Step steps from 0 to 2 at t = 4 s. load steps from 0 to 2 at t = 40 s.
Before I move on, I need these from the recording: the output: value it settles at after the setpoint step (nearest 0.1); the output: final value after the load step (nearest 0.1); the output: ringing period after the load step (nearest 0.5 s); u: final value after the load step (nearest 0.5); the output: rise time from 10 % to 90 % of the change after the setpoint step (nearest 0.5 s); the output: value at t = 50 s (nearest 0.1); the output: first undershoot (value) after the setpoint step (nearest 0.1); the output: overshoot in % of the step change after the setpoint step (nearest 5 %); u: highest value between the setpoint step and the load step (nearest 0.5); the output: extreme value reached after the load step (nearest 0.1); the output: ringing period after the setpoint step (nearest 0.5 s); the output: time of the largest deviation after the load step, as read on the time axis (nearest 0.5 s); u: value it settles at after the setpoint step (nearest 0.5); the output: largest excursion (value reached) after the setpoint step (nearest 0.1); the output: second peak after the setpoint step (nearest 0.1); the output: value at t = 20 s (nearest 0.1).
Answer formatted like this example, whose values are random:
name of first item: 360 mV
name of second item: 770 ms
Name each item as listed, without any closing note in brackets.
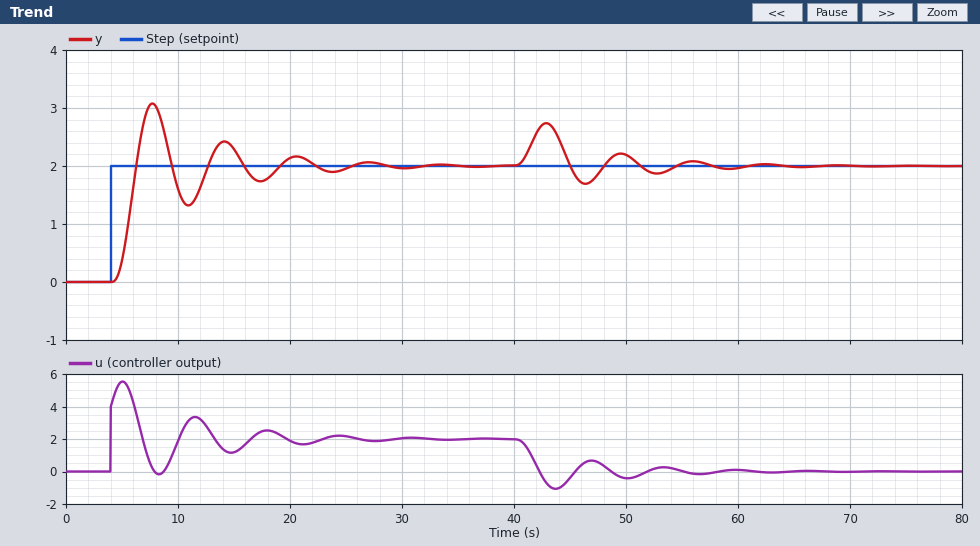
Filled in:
the output: value it settles at after the setpoint step: 2.0
the output: final value after the load step: 2.0
the output: ringing period after the load step: 6.5 s
u: final value after the load step: 0.0
the output: rise time from 10 % to 90 % of the change after the setpoint step: 1.5 s
the output: value at t = 50 s: 2.2
the output: first undershoot (value) after the setpoint step: 1.3
the output: overshoot in % of the step change after the setpoint step: 55 %
u: highest value between the setpoint step and the load step: 5.5
the output: extreme value reached after the load step: 2.7
the output: ringing period after the setpoint step: 6.5 s
the output: time of the largest deviation after the load step, as read on the time axis: 43.0 s
u: value it settles at after the setpoint step: 2.0
the output: largest excursion (value reached) after the setpoint step: 3.1
the output: second peak after the setpoint step: 2.4
the output: value at t = 20 s: 2.1
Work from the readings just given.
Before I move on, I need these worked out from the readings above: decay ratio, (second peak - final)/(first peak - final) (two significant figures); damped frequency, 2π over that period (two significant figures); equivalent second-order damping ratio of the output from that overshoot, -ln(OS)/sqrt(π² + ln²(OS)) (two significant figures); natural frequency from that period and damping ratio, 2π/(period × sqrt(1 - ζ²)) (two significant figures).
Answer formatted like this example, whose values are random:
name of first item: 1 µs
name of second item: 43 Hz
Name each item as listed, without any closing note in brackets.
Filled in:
decay ratio, (second peak - final)/(first peak - final): 0.36
damped frequency, 2π over that period: 0.97 rad/s
equivalent second-order damping ratio of the output from that overshoot, -ln(OS)/sqrt(π² + ln²(OS)): 0.19
natural frequency from that period and damping ratio, 2π/(period × sqrt(1 - ζ²)): 0.98 rad/s
